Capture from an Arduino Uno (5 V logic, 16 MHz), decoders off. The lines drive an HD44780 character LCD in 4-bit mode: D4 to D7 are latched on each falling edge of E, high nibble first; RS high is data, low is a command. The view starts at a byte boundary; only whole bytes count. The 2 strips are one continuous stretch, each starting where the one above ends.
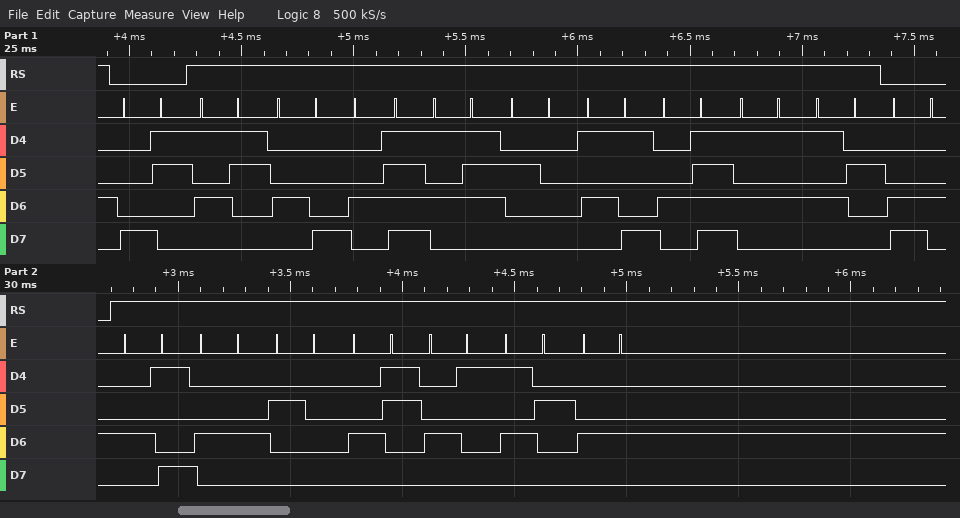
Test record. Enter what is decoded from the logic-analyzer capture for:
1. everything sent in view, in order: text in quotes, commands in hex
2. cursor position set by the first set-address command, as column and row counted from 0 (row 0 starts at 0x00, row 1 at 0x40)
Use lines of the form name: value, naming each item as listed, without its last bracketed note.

everything sent in view, in order: text in quotes, commands in hex: 0x83 "SHOW YOUR" 0xC4 "ID CARD"
cursor position set by the first set-address command, as column and row counted from 0: column 3, row 0
